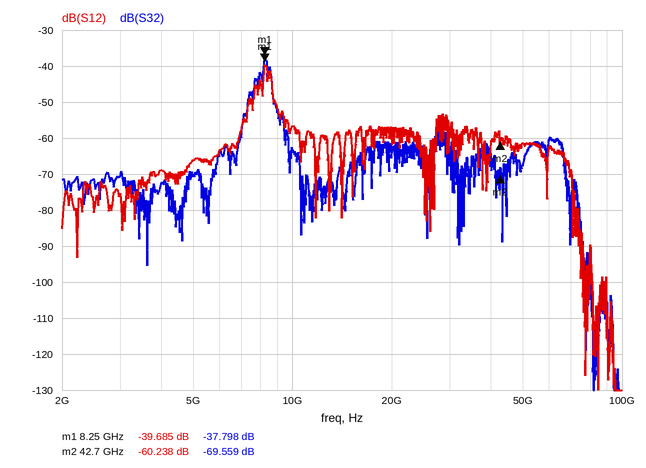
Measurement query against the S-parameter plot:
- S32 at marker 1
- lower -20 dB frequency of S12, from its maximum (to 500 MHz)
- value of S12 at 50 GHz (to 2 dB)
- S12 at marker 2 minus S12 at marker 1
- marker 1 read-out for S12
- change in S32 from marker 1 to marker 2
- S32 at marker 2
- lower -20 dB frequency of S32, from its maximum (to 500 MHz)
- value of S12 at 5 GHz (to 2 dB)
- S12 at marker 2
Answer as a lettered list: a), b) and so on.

a) -37.798 dB
b) 7.0 GHz
c) -62 dB
d) -20.553 dB
e) -39.685 dB
f) -31.761 dB
g) -69.559 dB
h) 7.0 GHz
i) -66 dB
j) -60.238 dB
